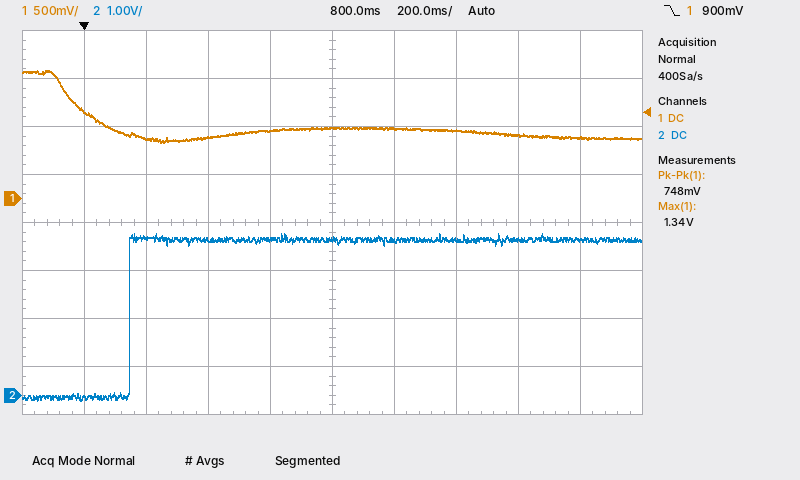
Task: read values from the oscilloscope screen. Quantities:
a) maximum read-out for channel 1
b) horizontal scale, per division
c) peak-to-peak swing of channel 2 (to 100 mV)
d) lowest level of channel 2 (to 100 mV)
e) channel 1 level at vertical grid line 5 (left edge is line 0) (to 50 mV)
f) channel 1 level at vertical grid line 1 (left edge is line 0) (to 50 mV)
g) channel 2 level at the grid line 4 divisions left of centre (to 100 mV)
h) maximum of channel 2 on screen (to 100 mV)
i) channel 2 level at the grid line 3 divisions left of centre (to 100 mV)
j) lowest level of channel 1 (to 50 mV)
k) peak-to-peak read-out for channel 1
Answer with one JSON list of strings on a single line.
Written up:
["1.34 V", "200 ms", "3.5 V", "-100 mV", "750 mV", "900 mV", "-100 mV", "3.4 V", "3.3 V", "600 mV", "748 mV"]
